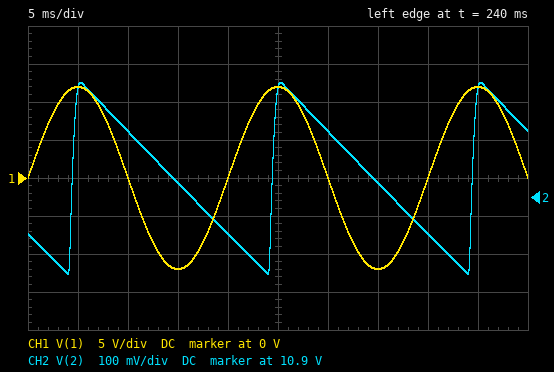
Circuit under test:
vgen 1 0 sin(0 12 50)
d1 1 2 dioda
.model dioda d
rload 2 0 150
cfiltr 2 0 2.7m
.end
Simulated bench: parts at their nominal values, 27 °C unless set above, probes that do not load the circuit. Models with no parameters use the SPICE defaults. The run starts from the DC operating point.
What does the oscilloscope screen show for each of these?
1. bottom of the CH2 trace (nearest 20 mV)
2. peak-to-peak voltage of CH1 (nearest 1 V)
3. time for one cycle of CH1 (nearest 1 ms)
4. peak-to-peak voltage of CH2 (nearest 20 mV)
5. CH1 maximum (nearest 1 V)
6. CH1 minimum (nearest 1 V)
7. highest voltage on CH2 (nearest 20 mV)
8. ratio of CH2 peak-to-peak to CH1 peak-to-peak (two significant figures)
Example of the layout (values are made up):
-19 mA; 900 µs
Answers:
10.70 V; 24 V; 20 ms; 500 mV; 12 V; -12 V; 11.20 V; 0.021
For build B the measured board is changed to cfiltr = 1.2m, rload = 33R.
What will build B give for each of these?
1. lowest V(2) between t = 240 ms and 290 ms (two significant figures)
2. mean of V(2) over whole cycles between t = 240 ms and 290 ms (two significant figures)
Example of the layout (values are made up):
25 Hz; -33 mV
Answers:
7.3 V; 9.2 V
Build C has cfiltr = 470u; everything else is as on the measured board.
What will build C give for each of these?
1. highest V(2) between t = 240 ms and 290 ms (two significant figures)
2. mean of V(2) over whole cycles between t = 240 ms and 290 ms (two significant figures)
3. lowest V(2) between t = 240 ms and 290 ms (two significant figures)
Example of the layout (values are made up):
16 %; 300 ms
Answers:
11 V; 10 V; 8.7 V
